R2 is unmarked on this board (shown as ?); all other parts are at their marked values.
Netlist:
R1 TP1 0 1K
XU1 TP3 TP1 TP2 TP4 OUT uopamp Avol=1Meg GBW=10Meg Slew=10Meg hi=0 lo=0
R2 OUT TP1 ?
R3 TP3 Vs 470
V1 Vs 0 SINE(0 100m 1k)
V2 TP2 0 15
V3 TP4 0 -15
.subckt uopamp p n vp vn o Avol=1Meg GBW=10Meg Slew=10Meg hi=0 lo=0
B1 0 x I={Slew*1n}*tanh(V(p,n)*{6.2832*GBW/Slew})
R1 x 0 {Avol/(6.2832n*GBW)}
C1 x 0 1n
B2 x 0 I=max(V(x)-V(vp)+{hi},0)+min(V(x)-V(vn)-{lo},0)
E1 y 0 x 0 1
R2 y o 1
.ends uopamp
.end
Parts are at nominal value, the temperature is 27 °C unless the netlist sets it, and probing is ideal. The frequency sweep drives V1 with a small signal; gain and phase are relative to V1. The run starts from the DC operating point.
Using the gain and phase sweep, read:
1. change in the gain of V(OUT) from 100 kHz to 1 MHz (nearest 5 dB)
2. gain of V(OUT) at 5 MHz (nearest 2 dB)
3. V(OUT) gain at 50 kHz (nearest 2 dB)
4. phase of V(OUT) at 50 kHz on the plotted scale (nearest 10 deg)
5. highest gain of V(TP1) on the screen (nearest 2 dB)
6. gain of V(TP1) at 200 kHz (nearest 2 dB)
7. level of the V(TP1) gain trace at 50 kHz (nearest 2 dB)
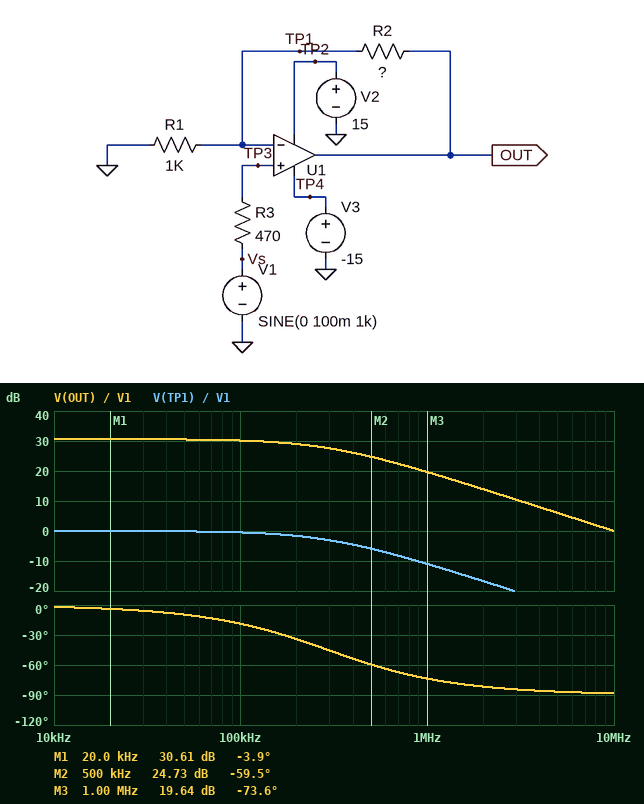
-10 dB
6 dB
30 dB
-10 deg
0 dB
-2 dB
0 dB
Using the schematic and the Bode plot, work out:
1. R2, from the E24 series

33 kΩ
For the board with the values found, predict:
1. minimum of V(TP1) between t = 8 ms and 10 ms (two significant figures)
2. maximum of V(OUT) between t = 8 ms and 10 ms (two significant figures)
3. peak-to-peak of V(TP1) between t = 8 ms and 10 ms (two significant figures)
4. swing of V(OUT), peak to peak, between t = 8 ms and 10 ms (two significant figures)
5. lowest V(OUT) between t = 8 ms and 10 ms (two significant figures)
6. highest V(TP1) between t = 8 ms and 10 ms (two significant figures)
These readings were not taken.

-100 mV
3.4 V
200 mV
6.8 V
-3.4 V
100 mV
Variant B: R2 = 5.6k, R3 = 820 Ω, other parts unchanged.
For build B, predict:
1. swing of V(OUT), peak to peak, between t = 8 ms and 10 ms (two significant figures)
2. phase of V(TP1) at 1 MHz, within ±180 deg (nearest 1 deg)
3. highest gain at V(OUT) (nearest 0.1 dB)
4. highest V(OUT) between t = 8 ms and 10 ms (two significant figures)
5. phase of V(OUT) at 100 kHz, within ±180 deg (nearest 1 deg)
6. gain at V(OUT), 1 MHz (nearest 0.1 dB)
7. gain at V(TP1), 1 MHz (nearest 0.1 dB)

1.3 V
-33 deg
16.4 dB
660 mV
-4 deg
14.8 dB
-1.6 dB
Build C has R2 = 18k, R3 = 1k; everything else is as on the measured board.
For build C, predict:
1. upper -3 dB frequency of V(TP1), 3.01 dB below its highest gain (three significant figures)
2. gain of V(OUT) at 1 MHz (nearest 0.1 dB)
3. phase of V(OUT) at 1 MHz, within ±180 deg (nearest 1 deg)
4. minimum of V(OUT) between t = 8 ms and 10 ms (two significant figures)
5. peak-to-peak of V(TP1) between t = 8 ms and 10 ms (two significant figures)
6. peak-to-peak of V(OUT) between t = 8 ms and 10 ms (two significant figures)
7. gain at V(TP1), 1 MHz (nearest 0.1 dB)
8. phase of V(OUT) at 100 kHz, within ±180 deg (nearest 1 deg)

526 kHz
18.9 dB
-62 deg
-1.9 V
200 mV
3.8 V
-6.6 dB
-11 deg
